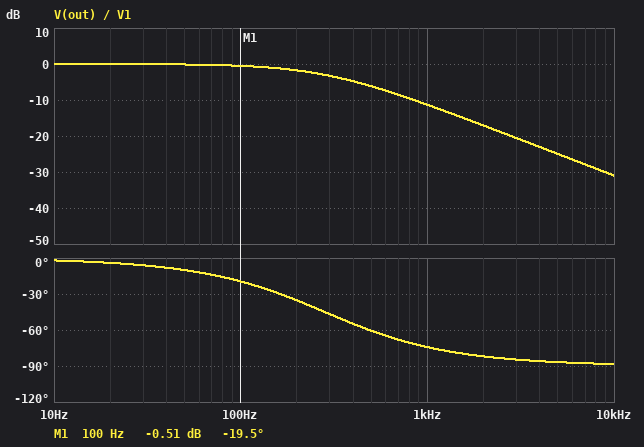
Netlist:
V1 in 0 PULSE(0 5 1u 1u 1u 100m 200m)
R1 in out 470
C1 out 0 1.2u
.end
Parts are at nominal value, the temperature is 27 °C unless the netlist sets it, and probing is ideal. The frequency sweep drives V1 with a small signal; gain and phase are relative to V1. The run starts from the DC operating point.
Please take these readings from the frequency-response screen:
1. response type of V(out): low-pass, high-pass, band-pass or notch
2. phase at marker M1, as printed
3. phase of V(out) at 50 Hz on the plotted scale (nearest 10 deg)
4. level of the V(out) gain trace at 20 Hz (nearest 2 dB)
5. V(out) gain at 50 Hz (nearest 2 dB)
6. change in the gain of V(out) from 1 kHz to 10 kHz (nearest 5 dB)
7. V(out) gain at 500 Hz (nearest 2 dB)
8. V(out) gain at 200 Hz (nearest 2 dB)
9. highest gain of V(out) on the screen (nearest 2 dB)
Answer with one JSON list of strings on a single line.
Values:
["low-pass", "-19.5 deg", "-10 deg", "0 dB", "0 dB", "-20 dB", "-6 dB", "-2 dB", "0 dB"]
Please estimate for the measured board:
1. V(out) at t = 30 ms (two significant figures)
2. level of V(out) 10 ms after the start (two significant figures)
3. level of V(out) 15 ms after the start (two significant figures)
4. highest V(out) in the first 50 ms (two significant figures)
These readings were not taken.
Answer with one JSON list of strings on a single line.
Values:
["5.0 V", "5.0 V", "5.0 V", "5.0 V"]
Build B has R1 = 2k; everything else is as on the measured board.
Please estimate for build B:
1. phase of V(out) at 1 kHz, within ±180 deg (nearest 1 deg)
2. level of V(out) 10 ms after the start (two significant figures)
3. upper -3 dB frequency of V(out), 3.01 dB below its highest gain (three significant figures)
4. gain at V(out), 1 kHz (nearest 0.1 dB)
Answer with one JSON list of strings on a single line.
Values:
["-86 deg", "4.9 V", "66.3 Hz", "-23.6 dB"]
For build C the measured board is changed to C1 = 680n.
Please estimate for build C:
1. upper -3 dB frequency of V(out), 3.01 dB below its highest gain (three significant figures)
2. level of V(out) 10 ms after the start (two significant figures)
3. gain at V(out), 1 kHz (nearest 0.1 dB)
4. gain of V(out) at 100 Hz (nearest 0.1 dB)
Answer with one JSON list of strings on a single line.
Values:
["498 Hz", "5.0 V", "-7.0 dB", "-0.2 dB"]
